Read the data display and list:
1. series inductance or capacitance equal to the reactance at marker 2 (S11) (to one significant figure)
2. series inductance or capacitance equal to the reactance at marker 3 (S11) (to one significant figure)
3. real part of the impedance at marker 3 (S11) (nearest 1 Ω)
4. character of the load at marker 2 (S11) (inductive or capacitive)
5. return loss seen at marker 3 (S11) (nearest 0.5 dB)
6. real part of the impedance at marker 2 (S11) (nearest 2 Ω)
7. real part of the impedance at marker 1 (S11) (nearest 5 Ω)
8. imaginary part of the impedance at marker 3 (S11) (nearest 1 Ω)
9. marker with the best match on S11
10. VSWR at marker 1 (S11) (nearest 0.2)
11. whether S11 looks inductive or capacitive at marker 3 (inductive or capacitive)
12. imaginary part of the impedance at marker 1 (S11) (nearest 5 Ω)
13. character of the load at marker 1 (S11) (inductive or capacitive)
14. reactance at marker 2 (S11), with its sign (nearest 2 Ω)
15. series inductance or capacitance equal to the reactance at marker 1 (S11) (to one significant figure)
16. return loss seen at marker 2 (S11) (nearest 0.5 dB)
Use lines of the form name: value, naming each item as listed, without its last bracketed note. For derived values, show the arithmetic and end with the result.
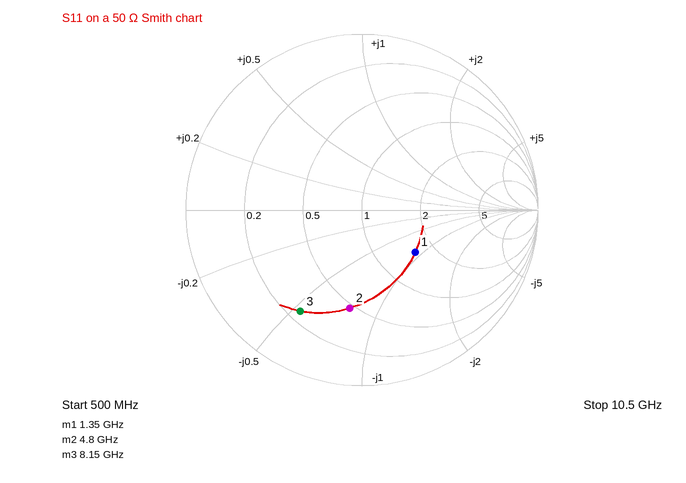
series inductance or capacitance equal to the reactance at marker 2 (S11): C = 1/(2π × 4.8 GHz × 38 Ω) ≈ 873 fF, so 900 fF to one significant figure
series inductance or capacitance equal to the reactance at marker 3 (S11): C = 1/(2π × 8.15 GHz × 27 Ω) ≈ 723 fF, so 700 fF to one significant figure
real part of the impedance at marker 3 (S11): 13 Ω
character of the load at marker 2 (S11): capacitive
return loss seen at marker 3 (S11): 3.5 dB
real part of the impedance at marker 2 (S11): 24 Ω
real part of the impedance at marker 1 (S11): 80 Ω
imaginary part of the impedance at marker 3 (S11): -27 Ω
marker with the best match on S11: marker 1
VSWR at marker 1 (S11): 2.2
whether S11 looks inductive or capacitive at marker 3: capacitive
imaginary part of the impedance at marker 1 (S11): -45 Ω
character of the load at marker 1 (S11): capacitive
reactance at marker 2 (S11), with its sign: -38 Ω
series inductance or capacitance equal to the reactance at marker 1 (S11): C = 1/(2π × 1.35 GHz × 45 Ω) ≈ 3 pF
return loss seen at marker 2 (S11): 5.0 dB
